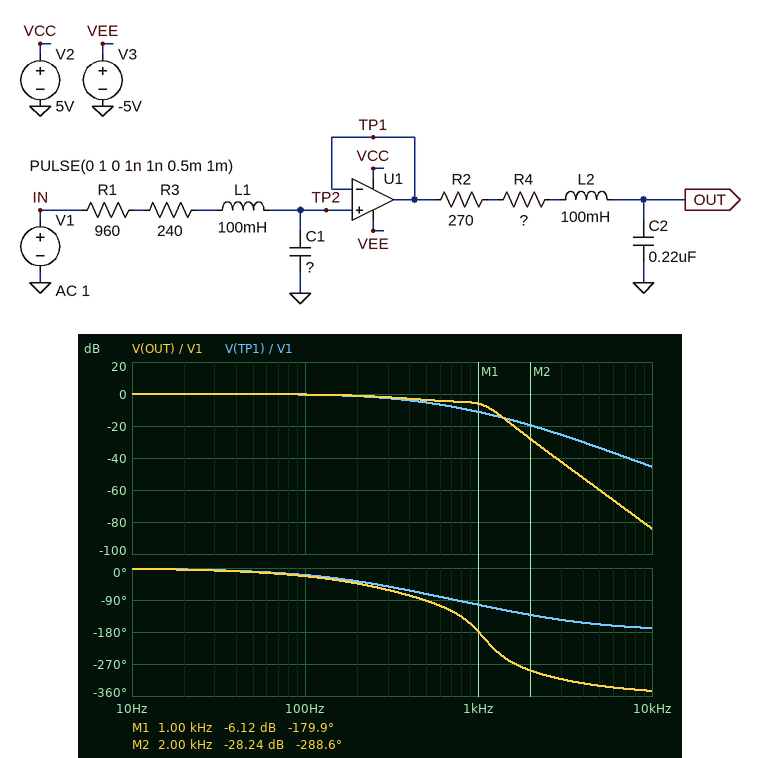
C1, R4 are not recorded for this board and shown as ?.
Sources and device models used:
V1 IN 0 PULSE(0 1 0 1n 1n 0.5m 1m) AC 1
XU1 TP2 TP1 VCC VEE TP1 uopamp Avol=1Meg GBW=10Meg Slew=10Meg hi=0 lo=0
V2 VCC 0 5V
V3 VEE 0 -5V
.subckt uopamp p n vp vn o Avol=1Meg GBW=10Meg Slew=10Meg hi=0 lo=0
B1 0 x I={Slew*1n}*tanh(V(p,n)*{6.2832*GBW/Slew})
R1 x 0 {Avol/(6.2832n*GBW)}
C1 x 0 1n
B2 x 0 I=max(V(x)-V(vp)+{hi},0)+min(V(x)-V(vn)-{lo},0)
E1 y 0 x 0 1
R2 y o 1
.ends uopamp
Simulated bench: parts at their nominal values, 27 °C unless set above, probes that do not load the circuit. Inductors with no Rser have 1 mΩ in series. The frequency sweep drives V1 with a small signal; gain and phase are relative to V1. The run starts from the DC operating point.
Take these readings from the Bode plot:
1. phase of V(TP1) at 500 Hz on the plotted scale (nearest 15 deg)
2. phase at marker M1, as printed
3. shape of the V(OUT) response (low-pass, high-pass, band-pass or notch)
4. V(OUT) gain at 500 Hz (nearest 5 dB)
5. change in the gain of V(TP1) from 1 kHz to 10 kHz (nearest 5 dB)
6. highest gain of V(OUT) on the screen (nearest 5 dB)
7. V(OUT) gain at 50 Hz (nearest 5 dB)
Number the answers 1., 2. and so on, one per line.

1. -75 deg
2. -179.9 deg
3. low-pass
4. -5 dB
5. -35 dB
6. 0 dB
7. 0 dB
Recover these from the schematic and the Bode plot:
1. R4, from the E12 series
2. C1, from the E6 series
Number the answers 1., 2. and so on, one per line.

1. 120 Ω
2. 470 nF
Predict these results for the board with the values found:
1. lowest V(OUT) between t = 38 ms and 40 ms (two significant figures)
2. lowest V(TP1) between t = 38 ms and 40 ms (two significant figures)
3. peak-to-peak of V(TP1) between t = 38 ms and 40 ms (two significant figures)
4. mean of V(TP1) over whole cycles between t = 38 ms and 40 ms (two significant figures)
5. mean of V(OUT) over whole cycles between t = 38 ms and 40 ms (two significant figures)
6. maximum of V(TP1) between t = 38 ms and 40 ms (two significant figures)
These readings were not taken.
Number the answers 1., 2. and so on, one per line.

1. 180 mV
2. 310 mV
3. 380 mV
4. 500 mV
5. 500 mV
6. 690 mV
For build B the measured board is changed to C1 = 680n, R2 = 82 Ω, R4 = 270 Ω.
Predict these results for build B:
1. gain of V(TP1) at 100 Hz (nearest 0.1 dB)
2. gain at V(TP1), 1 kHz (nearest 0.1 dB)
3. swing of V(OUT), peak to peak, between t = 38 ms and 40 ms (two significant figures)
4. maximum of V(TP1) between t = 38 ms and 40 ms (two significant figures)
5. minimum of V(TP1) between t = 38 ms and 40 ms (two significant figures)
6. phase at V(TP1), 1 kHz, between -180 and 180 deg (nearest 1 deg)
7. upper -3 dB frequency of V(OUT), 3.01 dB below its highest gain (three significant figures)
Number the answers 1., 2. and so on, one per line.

1. -0.8 dB
2. -14.6 dB
3. 470 mV
4. 630 mV
5. 370 mV
6. -108 deg
7. 235 Hz
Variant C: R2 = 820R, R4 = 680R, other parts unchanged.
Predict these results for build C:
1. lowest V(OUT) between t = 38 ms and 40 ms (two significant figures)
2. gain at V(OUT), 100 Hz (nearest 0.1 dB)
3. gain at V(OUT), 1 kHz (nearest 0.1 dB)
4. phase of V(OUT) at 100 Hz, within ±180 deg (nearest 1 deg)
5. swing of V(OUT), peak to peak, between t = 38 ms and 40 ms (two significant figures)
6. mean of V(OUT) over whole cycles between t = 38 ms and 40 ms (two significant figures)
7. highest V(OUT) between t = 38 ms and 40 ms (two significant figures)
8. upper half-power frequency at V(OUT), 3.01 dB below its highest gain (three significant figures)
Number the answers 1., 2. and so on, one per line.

1. 420 mV
2. -0.5 dB
3. -17.6 dB
4. -32 deg
5. 170 mV
6. 500 mV
7. 580 mV
8. 272 Hz
